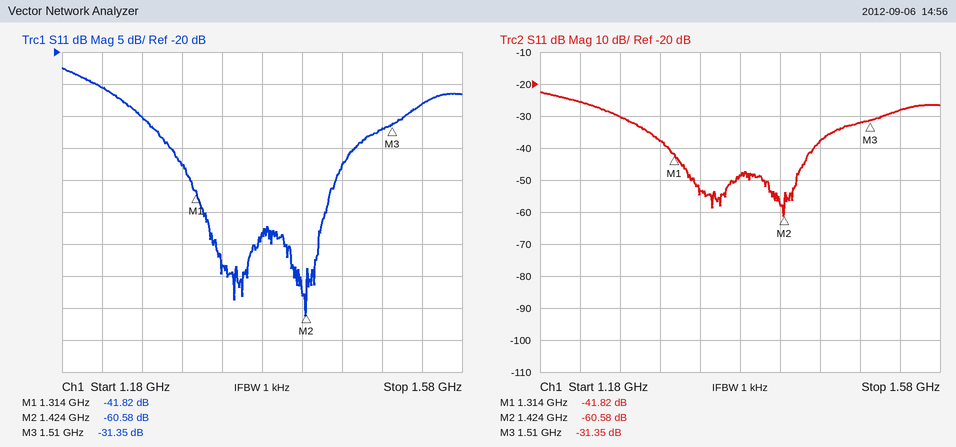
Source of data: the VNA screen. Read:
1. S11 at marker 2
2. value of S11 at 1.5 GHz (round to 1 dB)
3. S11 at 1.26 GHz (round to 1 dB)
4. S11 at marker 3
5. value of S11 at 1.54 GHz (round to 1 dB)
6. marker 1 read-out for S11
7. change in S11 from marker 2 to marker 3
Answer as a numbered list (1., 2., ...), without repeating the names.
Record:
1. -60.58 dB
2. -32 dB
3. -30 dB
4. -31.35 dB
5. -28 dB
6. -41.82 dB
7. 29.23 dB
